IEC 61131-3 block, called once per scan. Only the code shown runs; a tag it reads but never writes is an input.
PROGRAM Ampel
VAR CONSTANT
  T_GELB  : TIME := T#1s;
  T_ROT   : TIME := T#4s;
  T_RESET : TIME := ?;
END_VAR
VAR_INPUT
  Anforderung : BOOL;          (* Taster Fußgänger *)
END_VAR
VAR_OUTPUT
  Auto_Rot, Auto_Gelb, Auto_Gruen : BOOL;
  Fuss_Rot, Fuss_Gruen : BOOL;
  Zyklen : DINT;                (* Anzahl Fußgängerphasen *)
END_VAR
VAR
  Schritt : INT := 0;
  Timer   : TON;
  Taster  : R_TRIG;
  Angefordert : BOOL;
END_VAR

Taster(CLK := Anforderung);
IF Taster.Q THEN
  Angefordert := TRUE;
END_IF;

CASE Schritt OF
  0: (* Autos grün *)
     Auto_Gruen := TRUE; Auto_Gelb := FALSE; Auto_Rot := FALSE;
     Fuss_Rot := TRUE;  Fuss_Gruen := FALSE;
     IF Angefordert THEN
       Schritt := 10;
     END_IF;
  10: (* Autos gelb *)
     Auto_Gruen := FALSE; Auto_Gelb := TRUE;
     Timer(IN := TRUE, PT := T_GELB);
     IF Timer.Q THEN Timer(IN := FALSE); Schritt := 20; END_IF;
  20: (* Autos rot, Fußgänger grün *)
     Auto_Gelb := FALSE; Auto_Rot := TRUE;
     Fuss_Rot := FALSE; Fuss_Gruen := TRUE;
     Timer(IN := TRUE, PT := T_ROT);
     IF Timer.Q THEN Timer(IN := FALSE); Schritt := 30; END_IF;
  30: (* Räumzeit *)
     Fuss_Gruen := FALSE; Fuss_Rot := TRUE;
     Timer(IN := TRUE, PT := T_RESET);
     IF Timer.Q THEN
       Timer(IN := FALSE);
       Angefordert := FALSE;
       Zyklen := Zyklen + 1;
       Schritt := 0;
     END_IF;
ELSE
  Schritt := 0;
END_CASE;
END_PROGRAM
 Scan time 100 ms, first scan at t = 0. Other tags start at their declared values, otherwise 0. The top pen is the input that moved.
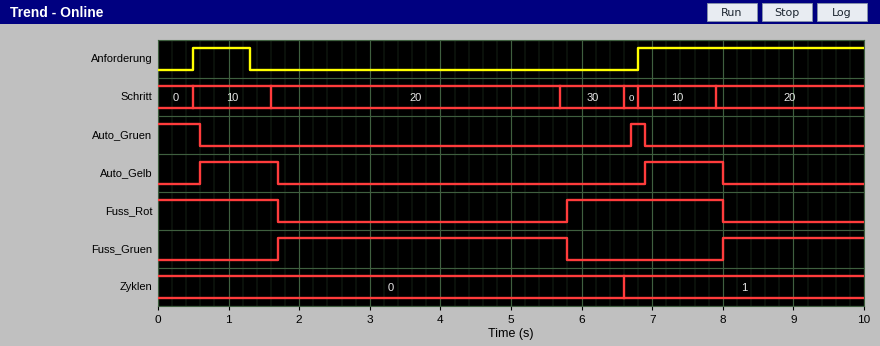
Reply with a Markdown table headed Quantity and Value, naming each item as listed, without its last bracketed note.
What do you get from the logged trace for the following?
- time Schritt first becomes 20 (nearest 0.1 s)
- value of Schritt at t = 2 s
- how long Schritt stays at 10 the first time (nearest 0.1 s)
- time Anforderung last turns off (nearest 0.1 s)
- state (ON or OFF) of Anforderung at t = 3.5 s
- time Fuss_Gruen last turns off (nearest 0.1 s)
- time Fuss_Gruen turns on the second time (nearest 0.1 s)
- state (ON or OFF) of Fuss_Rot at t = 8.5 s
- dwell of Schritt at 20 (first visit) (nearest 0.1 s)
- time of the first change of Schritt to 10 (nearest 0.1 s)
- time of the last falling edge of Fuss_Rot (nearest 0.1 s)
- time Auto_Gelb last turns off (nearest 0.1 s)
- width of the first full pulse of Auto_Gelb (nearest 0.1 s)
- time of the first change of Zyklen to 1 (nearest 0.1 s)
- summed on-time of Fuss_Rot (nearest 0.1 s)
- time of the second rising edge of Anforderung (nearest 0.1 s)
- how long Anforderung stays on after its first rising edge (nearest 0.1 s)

| Quantity | Value |
|---|---|
| time Schritt first becomes 20 | 1.6 s |
| value of Schritt at t = 2 s | 20 |
| how long Schritt stays at 10 the first time | 1.1 s |
| time Anforderung last turns off | 1.3 s |
| state (ON or OFF) of Anforderung at t = 3.5 s | OFF |
| time Fuss_Gruen last turns off | 5.8 s |
| time Fuss_Gruen turns on the second time | 8.0 s |
| state (ON or OFF) of Fuss_Rot at t = 8.5 s | OFF |
| dwell of Schritt at 20 (first visit) | 4.1 s |
| time of the first change of Schritt to 10 | 0.5 s |
| time of the last falling edge of Fuss_Rot | 8.0 s |
| time Auto_Gelb last turns off | 8.0 s |
| width of the first full pulse of Auto_Gelb | 1.1 s |
| time of the first change of Zyklen to 1 | 6.6 s |
| summed on-time of Fuss_Rot | 3.9 s |
| time of the second rising edge of Anforderung | 6.8 s |
| how long Anforderung stays on after its first rising edge | 0.8 s |
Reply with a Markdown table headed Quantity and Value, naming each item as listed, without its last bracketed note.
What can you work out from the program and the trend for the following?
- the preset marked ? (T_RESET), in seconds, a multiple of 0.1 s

| Quantity | Value |
|---|---|
| the preset marked ? (T_RESET), in seconds, a multiple of 0.1 s | 0.8 s |
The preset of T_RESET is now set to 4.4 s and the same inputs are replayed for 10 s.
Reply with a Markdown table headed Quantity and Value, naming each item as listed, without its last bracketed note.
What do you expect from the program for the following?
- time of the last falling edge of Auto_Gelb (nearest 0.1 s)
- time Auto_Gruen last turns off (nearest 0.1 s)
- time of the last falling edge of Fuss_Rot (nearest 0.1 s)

| Quantity | Value |
|---|---|
| time of the last falling edge of Auto_Gelb | 1.7 s |
| time Auto_Gruen last turns off | 0.6 s |
| time of the last falling edge of Fuss_Rot | 1.7 s |
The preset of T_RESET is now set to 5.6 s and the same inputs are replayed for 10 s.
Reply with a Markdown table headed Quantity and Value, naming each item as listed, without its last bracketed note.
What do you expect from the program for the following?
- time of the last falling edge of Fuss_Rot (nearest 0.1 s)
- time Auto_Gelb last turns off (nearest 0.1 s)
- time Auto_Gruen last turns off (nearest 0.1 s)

| Quantity | Value |
|---|---|
| time of the last falling edge of Fuss_Rot | 1.7 s |
| time Auto_Gelb last turns off | 1.7 s |
| time Auto_Gruen last turns off | 0.6 s |
